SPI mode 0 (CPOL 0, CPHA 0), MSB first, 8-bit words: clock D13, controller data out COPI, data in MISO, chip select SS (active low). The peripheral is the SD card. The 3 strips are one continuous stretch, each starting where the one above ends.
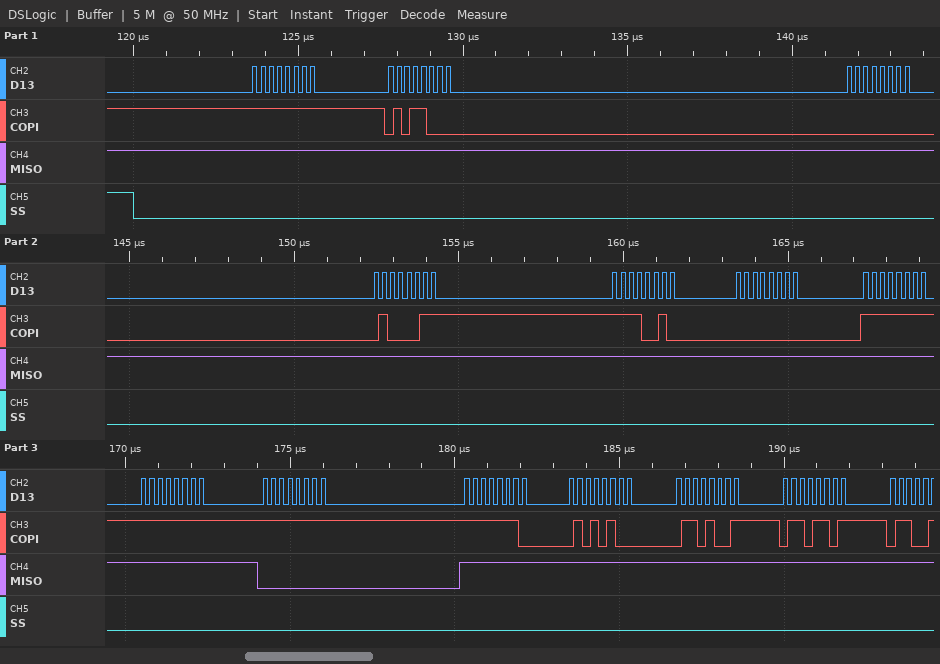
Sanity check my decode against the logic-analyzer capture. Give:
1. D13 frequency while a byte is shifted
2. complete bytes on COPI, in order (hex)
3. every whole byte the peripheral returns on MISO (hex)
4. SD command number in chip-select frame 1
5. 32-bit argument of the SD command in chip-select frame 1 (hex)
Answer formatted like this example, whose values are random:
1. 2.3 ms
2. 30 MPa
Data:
1. 4 MHz
2. 0xFF 0x58 0x00 0x43 0xF2 0x00 0xFF 0xFF 0xFF 0xFE 0x54 0x69 0x6D
3. 0xFF 0xFF 0xFF 0xFF 0xFF 0xFF 0xFF 0xFF 0x00 0xFF 0xFF 0xFF 0xFF
4. CMD24
5. 0x0043F200
